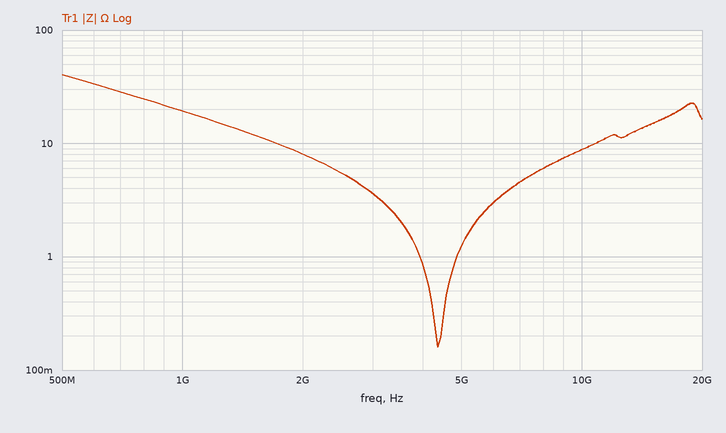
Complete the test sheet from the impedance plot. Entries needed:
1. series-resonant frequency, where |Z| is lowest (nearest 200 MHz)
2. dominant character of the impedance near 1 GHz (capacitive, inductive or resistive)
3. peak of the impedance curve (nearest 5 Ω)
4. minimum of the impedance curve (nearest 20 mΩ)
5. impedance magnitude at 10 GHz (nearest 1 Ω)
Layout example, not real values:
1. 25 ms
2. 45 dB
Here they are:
1. 4.4 GHz
2. capacitive
3. 40 Ω
4. 160 mΩ
5. 9 Ω
